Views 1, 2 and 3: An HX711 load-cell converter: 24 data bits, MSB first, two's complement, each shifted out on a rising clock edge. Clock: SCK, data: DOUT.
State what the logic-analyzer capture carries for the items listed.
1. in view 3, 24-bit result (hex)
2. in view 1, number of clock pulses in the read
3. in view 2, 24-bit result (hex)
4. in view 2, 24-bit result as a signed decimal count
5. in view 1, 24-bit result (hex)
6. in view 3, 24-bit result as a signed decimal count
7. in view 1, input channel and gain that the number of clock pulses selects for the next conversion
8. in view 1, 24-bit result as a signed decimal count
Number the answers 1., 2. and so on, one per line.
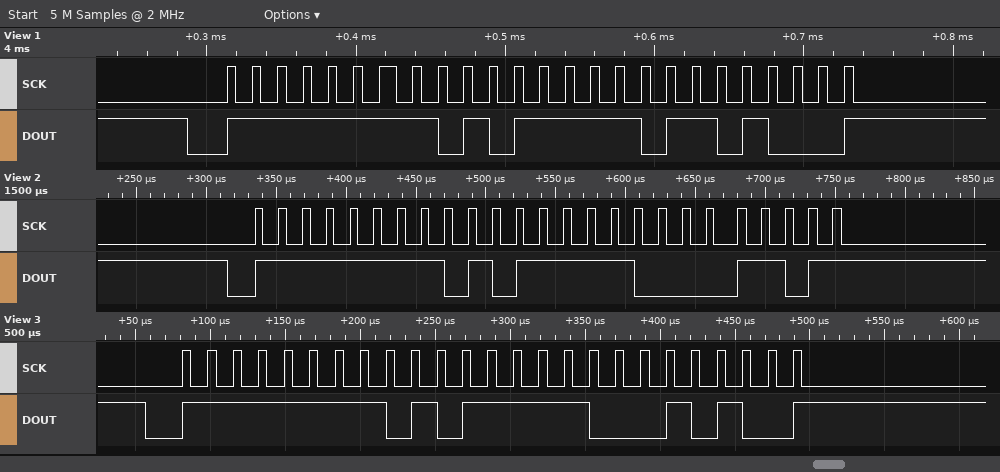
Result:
1. 0xFF5F14
2. 25
3. 0xFF5F0D
4. -41203
5. 0xFF5F68
6. -41196
7. channel A, gain 128
8. -41112
